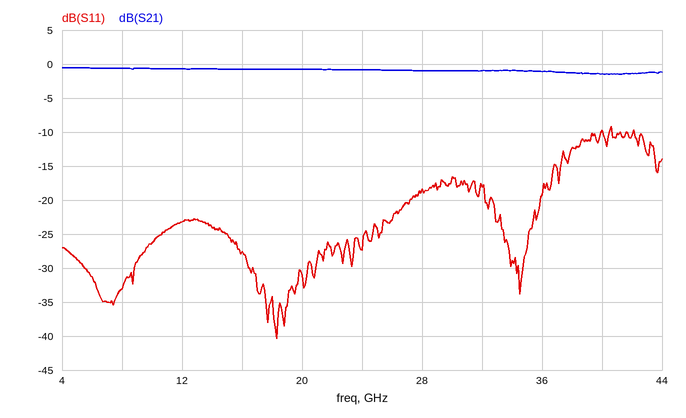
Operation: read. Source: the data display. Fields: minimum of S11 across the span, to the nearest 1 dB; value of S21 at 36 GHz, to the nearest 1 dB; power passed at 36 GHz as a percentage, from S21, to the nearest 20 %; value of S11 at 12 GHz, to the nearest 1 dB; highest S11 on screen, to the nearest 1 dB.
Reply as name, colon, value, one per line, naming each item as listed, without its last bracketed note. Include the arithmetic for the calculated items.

minimum of S11 across the span, to the nearest 1 dB: -40 dB
value of S21 at 36 GHz, to the nearest 1 dB: -1 dB
power passed at 36 GHz as a percentage, from S21, to the nearest 20 %: 10^(-1/10) ≈ 79.4 %, so 80 % to the nearest 20 %
value of S11 at 12 GHz, to the nearest 1 dB: -23 dB
highest S11 on screen, to the nearest 1 dB: -9 dB
